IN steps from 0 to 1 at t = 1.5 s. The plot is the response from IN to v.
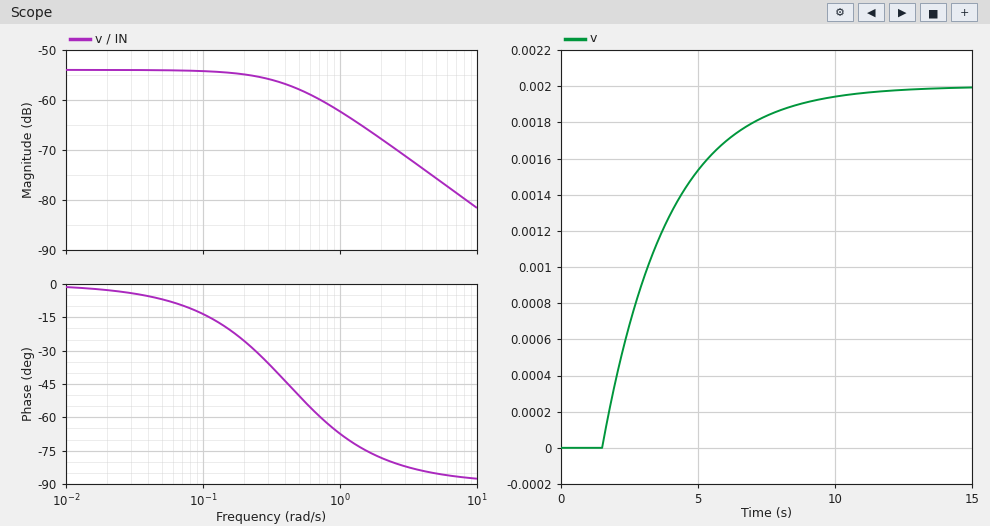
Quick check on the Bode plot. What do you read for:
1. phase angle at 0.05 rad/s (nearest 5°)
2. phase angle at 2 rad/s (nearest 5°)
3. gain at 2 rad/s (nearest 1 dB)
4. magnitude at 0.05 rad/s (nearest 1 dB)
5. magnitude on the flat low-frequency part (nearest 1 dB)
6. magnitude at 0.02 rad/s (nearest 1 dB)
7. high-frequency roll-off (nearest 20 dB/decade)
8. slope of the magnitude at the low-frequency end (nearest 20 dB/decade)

-5°
-80°
-68 dB
-54 dB
-54 dB
-54 dB
-20 dB/decade
0 dB/decade
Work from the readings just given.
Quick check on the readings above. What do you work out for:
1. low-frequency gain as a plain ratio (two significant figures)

0.0020
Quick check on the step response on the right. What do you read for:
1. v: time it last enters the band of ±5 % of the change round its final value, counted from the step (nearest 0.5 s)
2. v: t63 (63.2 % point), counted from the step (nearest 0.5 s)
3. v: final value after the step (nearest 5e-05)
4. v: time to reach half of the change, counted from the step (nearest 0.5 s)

7.0 s
2.5 s
0.00200
1.5 s
